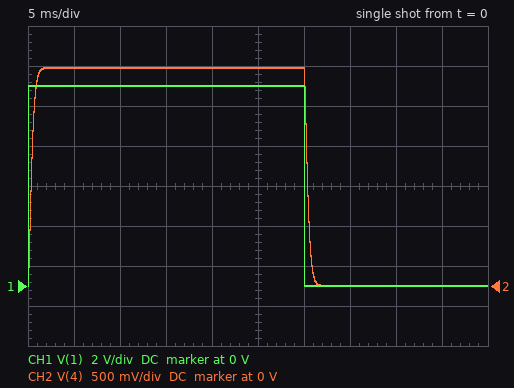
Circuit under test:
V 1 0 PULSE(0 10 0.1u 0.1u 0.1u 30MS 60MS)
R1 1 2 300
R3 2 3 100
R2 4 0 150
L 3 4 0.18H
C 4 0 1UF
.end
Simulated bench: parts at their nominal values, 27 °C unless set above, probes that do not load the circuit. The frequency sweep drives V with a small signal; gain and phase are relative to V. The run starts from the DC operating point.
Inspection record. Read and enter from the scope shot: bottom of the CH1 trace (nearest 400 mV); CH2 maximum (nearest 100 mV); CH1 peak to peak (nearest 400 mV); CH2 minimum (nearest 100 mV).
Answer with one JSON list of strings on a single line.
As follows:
["0 V", "2.7 V", "10.0 V", "0 V"]
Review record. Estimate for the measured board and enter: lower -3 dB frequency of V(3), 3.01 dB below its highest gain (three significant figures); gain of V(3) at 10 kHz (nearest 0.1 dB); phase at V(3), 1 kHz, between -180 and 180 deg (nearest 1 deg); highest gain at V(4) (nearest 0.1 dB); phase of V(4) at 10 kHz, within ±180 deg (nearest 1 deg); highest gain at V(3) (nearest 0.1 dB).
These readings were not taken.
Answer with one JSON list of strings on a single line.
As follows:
["487 Hz", "0 dB", "20 deg", "-11.3 dB", "-172 deg", "0 dB"]
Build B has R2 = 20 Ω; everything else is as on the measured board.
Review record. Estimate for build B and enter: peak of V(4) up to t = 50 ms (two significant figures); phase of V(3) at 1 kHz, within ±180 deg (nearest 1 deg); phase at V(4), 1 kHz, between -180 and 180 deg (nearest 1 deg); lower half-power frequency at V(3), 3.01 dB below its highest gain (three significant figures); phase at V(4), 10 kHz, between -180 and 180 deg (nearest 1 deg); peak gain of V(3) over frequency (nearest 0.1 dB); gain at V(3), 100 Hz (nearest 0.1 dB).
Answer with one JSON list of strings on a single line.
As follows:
["480 mV", "19 deg", "-77 deg", "371 Hz", "-139 deg", "0 dB", "-11.6 dB"]
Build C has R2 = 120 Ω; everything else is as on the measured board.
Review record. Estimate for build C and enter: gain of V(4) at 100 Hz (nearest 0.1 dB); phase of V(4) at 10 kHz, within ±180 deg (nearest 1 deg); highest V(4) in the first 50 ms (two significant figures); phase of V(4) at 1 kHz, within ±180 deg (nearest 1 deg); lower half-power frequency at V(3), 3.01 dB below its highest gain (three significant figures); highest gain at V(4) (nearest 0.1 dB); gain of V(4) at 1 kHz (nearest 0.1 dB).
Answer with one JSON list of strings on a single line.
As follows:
["-12.9 dB", "-170 deg", "2.3 V", "-103 deg", "461 Hz", "-12.7 dB", "-21.8 dB"]
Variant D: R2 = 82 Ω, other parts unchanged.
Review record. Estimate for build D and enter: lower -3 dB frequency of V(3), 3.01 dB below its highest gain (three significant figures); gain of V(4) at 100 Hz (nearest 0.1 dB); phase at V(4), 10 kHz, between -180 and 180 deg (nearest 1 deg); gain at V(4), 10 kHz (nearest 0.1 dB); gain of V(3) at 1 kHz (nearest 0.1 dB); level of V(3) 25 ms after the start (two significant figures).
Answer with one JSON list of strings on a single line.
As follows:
["427 Hz", "-15.6 dB", "-167 deg", "-57.2 dB", "-0.7 dB", "1.7 V"]
